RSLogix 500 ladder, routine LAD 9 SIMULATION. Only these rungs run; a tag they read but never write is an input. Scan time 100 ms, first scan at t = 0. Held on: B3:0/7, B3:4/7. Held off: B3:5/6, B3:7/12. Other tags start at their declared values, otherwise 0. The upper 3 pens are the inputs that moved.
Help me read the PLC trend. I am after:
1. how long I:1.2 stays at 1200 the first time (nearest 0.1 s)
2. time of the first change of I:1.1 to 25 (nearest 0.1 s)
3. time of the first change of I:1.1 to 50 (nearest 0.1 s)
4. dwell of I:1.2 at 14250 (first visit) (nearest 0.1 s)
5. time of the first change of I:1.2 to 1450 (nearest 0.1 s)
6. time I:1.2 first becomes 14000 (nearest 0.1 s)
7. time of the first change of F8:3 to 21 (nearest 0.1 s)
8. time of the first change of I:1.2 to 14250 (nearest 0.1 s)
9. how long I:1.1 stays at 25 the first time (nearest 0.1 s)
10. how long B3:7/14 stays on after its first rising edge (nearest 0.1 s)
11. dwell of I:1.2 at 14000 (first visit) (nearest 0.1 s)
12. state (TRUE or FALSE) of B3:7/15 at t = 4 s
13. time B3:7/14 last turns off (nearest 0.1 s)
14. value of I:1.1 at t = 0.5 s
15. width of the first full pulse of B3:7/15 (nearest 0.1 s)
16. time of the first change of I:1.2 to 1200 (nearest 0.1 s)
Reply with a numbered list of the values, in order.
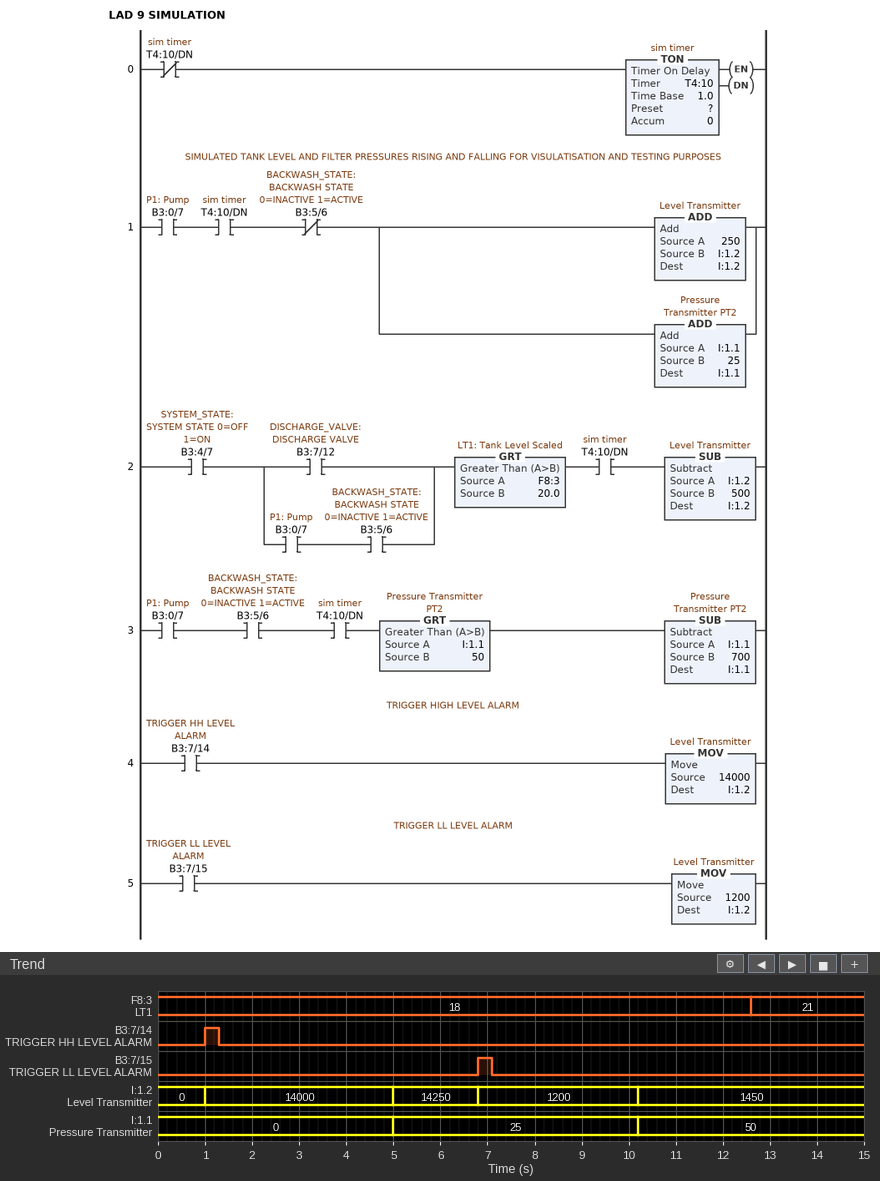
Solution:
1. 3.4 s
2. 5.0 s
3. 10.2 s
4. 1.8 s
5. 10.2 s
6. 1.0 s
7. 12.6 s
8. 5.0 s
9. 5.2 s
10. 0.3 s
11. 4.0 s
12. FALSE
13. 1.3 s
14. 0
15. 0.3 s
16. 6.8 s
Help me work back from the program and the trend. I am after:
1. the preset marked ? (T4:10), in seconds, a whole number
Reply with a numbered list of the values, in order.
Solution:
1. 5 s
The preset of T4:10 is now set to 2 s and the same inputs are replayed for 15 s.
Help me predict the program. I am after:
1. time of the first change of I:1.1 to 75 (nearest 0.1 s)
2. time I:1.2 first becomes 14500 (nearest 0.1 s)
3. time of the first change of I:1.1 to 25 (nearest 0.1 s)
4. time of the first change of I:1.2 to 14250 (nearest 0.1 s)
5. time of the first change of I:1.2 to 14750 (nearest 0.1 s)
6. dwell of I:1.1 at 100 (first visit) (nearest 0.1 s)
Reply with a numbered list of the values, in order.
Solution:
1. 6.4 s
2. 4.2 s
3. 2.0 s
4. 2.0 s
5. 6.4 s
6. 2.2 s
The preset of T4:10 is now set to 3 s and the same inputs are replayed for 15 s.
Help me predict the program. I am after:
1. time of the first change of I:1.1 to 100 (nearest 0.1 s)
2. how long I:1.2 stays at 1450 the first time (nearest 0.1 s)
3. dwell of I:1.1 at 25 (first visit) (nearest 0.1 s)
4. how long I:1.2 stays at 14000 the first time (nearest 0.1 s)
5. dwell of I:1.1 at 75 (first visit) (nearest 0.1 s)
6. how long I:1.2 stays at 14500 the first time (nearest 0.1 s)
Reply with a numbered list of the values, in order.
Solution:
1. 12.6 s
2. 3.2 s
3. 3.2 s
4. 2.0 s
5. 3.2 s
6. 0.6 s
